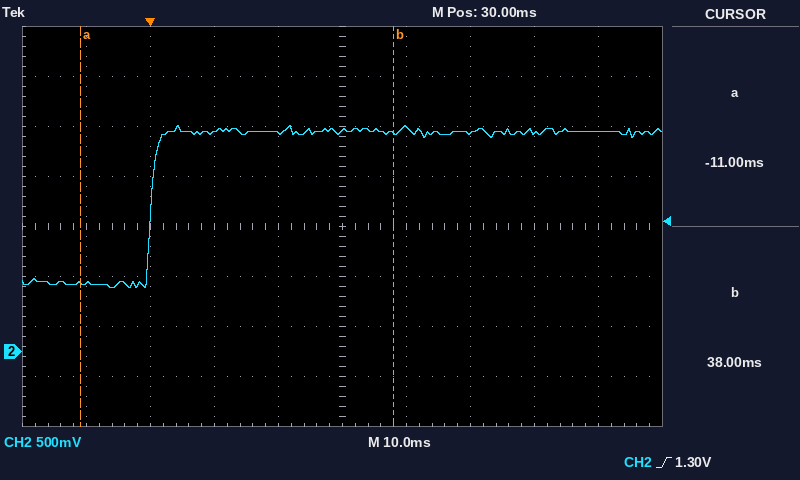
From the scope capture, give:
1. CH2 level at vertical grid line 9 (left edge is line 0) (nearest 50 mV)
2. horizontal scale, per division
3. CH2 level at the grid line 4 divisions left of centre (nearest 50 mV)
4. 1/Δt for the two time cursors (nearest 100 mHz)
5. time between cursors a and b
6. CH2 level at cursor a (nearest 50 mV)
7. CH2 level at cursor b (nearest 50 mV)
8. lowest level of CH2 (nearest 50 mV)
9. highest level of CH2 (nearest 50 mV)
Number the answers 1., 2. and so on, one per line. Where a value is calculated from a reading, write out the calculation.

1. 2.20 V
2. 10 ms
3. 700 mV
4. 1 / 49 ms ≈ 20.4 Hz
5. 38 ms − (-11 ms) = 49 ms
6. 700 mV
7. 2.20 V
8. 650 mV
9. 2.25 V
